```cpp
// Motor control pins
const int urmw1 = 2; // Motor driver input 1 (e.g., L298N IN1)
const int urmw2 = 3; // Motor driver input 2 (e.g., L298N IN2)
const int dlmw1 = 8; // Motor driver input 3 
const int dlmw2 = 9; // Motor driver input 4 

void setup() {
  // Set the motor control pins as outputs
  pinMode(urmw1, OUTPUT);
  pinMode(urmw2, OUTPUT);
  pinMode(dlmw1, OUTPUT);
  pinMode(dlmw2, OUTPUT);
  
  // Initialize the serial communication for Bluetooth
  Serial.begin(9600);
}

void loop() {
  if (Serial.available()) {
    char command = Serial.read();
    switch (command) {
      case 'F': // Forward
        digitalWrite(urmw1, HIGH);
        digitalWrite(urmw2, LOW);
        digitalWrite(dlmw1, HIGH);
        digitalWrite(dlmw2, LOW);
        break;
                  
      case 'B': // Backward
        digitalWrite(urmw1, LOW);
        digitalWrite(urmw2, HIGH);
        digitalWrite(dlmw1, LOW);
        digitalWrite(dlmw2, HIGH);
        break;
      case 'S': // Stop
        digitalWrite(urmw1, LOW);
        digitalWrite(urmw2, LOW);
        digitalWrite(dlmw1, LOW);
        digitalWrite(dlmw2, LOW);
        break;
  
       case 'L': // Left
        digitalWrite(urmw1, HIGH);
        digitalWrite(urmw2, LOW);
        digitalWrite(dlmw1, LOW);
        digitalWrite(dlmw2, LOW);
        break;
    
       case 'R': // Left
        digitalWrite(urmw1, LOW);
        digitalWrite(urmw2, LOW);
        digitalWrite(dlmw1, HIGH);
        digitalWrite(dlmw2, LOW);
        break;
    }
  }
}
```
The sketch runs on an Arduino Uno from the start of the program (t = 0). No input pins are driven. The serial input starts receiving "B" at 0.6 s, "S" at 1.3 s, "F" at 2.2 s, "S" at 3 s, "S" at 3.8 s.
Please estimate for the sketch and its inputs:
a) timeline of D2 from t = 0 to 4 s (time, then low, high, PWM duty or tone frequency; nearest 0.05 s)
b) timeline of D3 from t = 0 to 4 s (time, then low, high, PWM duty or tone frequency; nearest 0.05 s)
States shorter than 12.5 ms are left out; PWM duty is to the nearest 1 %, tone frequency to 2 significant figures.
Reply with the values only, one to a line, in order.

0 s low; 2.2 s high; 3 s low
0 s low; 0.6 s high; 1.3 s low
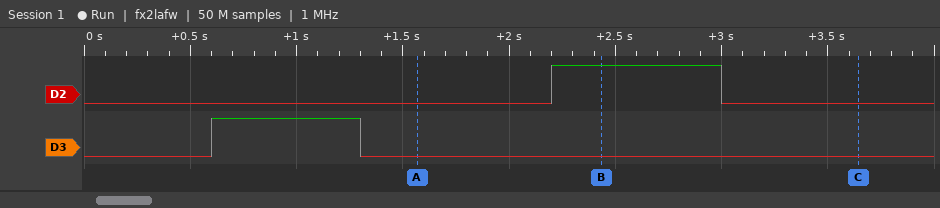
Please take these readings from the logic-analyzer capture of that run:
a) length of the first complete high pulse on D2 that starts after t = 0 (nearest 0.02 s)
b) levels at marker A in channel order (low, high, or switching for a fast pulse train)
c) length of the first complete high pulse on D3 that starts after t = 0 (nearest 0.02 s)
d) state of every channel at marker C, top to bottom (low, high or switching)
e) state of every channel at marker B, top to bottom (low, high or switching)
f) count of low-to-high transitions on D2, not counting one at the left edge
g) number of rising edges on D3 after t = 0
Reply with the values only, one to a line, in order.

0.80 s
D2 low, D3 low
0.70 s
D2 low, D3 low
D2 high, D3 low
1
1
